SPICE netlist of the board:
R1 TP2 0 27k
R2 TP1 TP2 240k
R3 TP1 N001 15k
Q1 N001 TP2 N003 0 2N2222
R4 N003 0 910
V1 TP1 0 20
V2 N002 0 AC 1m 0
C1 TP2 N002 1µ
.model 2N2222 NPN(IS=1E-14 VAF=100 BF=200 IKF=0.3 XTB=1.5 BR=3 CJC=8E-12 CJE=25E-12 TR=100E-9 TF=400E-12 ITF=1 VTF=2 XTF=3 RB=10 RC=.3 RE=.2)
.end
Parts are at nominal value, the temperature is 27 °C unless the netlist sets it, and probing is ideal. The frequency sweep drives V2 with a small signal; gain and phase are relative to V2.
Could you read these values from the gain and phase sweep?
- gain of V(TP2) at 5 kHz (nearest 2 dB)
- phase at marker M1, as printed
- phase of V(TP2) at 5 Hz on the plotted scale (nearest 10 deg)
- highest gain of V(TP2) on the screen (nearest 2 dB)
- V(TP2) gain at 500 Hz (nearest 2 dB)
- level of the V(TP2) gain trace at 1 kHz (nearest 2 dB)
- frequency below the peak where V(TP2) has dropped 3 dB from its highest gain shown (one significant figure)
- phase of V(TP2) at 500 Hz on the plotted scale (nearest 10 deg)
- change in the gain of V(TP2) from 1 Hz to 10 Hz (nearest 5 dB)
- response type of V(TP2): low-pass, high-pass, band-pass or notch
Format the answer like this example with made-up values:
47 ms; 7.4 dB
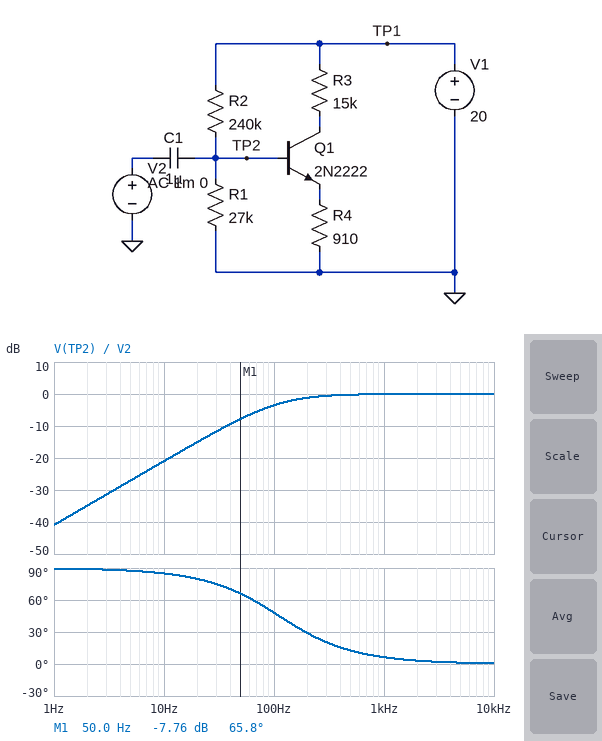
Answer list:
0 dB; 65.8 deg; 90 deg; 0 dB; 0 dB; 0 dB; 100 Hz; 10 deg; 20 dB; high-pass
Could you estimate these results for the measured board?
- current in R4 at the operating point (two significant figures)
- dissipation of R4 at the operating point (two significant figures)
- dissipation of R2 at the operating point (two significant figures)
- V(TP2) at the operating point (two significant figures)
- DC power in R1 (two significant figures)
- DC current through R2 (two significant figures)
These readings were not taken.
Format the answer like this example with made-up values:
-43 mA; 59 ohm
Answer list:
1.3 mA; 1.4 mW; 1.4 mW; 1.8 V; 120 µW; 76 µA
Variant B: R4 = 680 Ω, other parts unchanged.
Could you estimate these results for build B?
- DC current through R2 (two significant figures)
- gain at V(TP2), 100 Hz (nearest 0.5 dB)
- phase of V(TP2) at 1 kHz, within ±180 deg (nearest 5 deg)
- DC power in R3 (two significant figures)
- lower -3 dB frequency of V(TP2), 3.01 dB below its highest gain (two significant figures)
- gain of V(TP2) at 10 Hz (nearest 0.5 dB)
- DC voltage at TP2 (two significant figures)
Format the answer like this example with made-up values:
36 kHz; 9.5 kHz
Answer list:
77 µA; -7.0 dB; 10 deg; 24 mW; 200 Hz; -26.0 dB; 1.5 V
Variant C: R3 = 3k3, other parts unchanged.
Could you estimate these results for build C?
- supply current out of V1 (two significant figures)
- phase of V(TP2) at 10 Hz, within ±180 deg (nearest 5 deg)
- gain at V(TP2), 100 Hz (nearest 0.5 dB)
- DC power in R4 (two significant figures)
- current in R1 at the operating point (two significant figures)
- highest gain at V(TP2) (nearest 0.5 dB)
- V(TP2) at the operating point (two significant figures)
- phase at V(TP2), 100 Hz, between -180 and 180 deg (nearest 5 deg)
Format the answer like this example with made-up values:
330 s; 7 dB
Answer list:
1.4 mA; 35 deg; 0 dB; 1.6 mW; 70 µA; 0 dB; 1.9 V; 5 deg
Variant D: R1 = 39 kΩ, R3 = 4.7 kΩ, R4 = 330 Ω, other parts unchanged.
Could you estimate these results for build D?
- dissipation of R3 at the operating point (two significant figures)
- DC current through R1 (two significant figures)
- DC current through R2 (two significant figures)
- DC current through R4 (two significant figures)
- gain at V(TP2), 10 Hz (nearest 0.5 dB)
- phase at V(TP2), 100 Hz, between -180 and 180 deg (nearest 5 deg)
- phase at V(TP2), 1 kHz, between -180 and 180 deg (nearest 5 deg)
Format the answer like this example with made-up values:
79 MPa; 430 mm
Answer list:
73 mW; 51 µA; 75 µA; 4.0 mA; -26.0 dB; 65 deg; 10 deg
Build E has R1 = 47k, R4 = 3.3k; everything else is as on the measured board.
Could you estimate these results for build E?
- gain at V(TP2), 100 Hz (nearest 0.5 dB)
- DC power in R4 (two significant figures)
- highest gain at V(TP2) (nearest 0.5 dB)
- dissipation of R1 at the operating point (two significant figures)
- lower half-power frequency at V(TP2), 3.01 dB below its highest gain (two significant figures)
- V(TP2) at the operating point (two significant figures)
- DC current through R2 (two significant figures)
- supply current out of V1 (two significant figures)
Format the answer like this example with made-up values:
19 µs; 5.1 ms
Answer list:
0 dB; 1.9 mW; 0 dB; 210 µW; 4.3 Hz; 3.1 V; 70 µA; 820 µA
